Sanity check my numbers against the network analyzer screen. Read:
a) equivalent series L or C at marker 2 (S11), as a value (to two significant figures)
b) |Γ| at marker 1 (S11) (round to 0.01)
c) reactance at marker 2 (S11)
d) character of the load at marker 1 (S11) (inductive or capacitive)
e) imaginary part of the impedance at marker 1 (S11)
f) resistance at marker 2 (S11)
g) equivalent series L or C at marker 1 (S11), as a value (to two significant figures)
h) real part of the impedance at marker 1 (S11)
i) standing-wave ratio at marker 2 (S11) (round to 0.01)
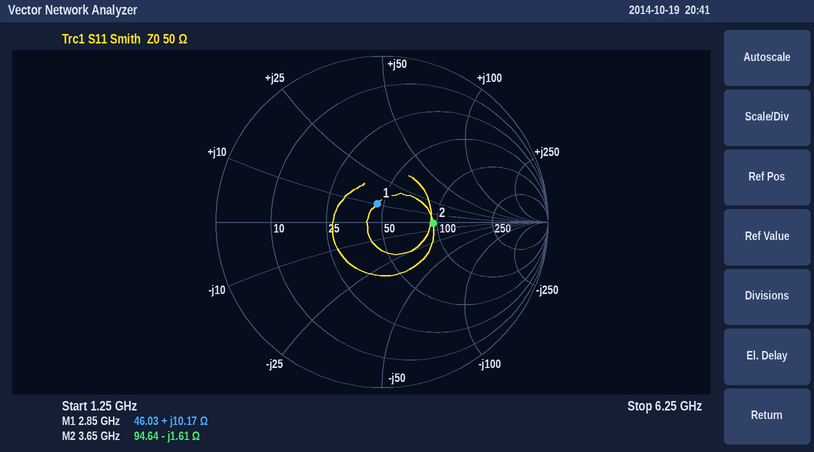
27 pF
0.11
-1.61 Ω
inductive
+10.17 Ω
94.64 Ω
570 pH
46.03 Ω
1.89
